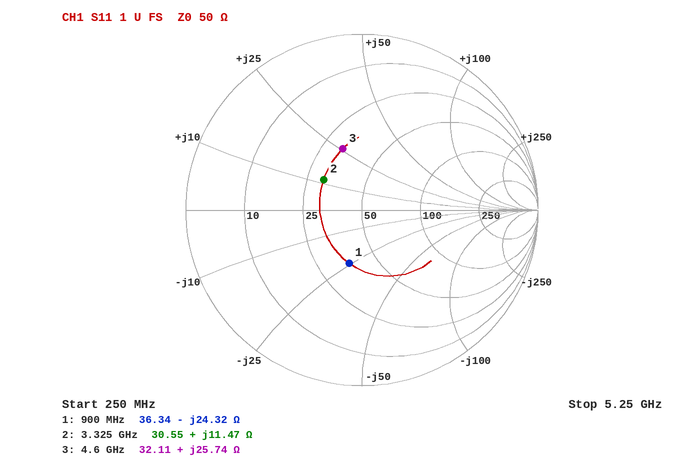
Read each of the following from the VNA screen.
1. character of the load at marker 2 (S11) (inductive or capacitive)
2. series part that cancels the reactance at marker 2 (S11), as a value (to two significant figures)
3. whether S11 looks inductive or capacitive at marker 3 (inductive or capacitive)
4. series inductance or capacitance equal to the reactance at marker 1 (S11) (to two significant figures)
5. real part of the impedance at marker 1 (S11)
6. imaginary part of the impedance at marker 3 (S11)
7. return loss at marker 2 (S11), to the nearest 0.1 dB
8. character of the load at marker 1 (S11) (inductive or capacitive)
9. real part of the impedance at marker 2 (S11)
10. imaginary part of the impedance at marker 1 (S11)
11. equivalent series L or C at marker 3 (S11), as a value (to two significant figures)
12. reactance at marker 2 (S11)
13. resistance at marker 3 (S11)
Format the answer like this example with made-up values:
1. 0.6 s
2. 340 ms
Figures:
1. inductive
2. 4.2 pF
3. inductive
4. 7.3 pF
5. 36.34 Ω
6. +25.74 Ω
7. 11.1 dB
8. capacitive
9. 30.55 Ω
10. -24.32 Ω
11. 890 pH
12. +11.47 Ω
13. 32.11 Ω
